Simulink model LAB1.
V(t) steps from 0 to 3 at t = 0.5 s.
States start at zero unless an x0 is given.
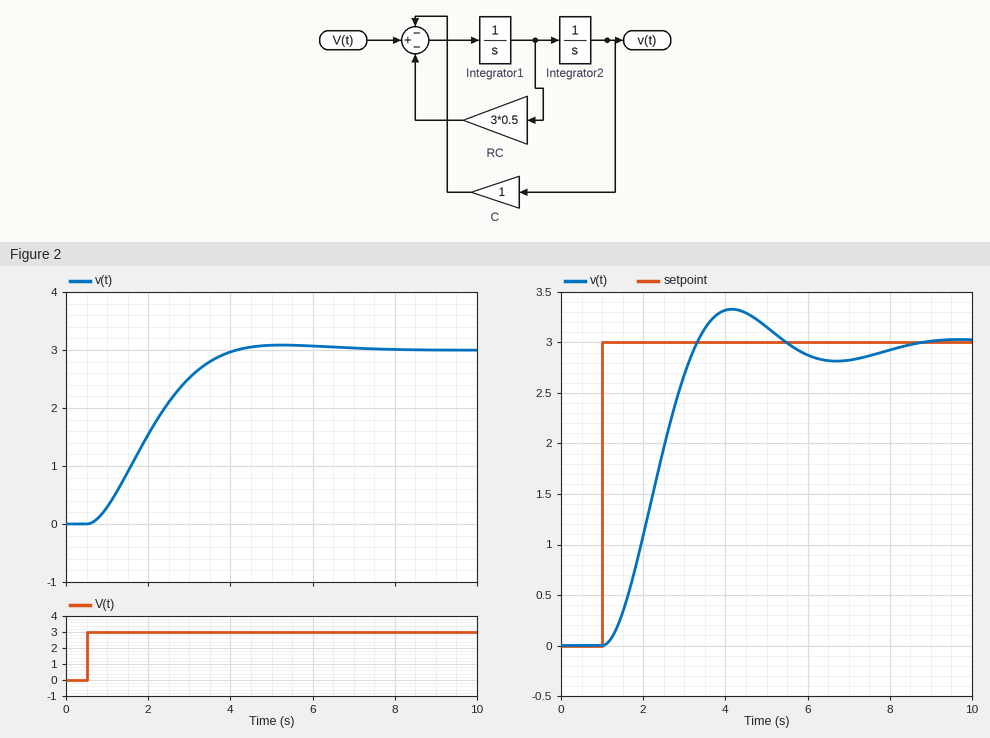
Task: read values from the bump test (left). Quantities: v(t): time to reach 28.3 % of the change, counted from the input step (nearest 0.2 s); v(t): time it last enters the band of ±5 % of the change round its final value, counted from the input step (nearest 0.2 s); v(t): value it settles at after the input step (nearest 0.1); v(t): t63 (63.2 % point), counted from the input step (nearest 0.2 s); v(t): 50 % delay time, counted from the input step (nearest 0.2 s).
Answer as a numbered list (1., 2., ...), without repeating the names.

1. 1.0 s
2. 3.2 s
3. 3.0
4. 1.8 s
5. 1.4 s
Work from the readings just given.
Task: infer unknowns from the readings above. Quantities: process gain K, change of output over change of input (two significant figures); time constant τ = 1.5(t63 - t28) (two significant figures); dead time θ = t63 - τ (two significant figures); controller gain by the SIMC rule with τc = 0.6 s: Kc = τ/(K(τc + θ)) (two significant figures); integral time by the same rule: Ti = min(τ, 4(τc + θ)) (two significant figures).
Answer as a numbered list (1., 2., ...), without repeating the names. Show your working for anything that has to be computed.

1. (3 - 0) / 3 = 1.0
2. 1.5 × (1.8 - 1) = 1.2 s
3. 1.8 - 1.2 = 0.60 s
4. 1.2 / (1 × (0.6 + 0.6)) = 1.0
5. min(1.2, 4 × (0.6 + 0.6)) = 1.2 s
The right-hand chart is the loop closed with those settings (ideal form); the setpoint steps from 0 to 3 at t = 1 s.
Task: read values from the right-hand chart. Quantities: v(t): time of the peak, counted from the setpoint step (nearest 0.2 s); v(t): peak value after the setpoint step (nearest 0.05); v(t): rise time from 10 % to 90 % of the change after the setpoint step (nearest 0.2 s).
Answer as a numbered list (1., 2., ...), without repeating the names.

1. 3.2 s
2. 3.35
3. 1.6 s
